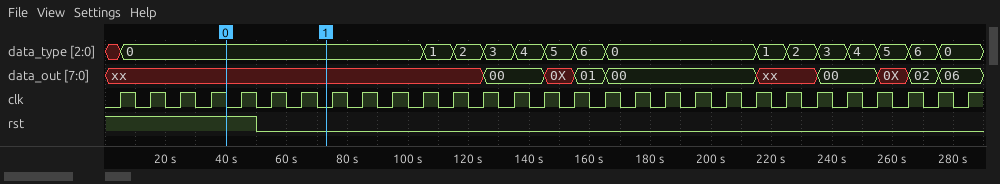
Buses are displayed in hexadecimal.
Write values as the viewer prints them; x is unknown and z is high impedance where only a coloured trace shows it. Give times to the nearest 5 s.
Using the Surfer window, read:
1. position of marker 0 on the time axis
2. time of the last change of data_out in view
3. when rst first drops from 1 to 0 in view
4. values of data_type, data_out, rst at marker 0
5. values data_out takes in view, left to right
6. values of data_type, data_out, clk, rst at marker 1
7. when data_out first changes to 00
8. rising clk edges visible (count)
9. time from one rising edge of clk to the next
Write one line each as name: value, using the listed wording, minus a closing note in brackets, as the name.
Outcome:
position of marker 0 on the time axis: 40 s
time of the last change of data_out in view: 275 s
when rst first drops from 1 to 0 in view: 50 s
values of data_type, data_out, rst at marker 0: data_type=0, data_out=xx, rst=1
values data_out takes in view, left to right: xx, 00, 0X, 01, 00, xx, 00, 0X, 02, 06
values of data_type, data_out, clk, rst at marker 1: data_type=0, data_out=xx, clk=0, rst=0
when data_out first changes to 00: 125 s
rising clk edges visible: 29
time from one rising edge of clk to the next: 10 s
